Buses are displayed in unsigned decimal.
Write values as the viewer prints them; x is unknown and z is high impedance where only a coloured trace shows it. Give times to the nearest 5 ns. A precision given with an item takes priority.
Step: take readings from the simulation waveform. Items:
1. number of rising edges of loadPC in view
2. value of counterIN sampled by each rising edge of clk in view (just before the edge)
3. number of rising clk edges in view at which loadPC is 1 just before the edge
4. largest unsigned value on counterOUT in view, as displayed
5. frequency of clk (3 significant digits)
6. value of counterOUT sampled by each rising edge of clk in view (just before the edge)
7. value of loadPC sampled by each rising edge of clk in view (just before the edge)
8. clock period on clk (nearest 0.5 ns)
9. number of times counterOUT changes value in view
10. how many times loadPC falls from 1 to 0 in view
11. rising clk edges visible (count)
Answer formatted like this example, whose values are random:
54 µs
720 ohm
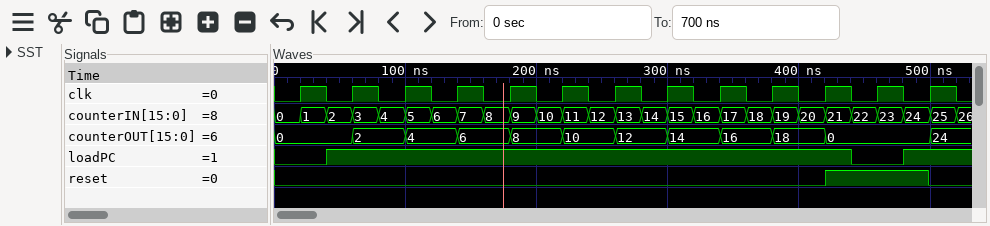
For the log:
2
0, 2, 4, 6, 8, 10, 12, 14, 16, 18, 20, 22, 24
11
24
25.0 MHz
0, 0, 2, 4, 6, 8, 10, 12, 14, 16, 18, 0, 0
0 1 1 1 1 1 1 1 1 1 1 0 1
40 ns
11
1
13
